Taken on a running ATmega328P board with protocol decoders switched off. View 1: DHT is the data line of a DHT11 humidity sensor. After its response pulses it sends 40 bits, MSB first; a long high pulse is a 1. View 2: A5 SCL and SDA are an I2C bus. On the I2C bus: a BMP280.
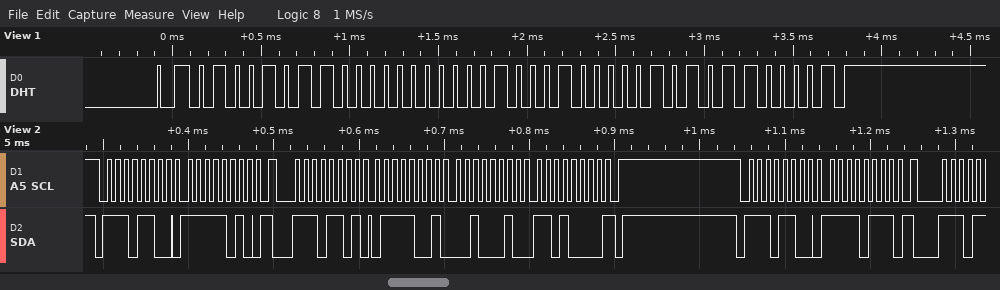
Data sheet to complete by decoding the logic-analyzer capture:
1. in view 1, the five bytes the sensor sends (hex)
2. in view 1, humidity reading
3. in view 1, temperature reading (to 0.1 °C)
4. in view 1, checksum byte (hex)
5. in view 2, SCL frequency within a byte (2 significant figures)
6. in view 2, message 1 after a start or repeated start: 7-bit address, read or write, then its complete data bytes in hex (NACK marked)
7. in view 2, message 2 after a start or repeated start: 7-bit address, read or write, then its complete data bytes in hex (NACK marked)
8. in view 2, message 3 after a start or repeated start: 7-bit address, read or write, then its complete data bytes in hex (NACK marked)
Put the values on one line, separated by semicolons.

4B 00 11 05 61; 75 %; 17.5 °C; 0x61; 100 kHz; 0x76 write: FA; 0x76 read: 79 22 D0 NACK; 0x76 write: F7
